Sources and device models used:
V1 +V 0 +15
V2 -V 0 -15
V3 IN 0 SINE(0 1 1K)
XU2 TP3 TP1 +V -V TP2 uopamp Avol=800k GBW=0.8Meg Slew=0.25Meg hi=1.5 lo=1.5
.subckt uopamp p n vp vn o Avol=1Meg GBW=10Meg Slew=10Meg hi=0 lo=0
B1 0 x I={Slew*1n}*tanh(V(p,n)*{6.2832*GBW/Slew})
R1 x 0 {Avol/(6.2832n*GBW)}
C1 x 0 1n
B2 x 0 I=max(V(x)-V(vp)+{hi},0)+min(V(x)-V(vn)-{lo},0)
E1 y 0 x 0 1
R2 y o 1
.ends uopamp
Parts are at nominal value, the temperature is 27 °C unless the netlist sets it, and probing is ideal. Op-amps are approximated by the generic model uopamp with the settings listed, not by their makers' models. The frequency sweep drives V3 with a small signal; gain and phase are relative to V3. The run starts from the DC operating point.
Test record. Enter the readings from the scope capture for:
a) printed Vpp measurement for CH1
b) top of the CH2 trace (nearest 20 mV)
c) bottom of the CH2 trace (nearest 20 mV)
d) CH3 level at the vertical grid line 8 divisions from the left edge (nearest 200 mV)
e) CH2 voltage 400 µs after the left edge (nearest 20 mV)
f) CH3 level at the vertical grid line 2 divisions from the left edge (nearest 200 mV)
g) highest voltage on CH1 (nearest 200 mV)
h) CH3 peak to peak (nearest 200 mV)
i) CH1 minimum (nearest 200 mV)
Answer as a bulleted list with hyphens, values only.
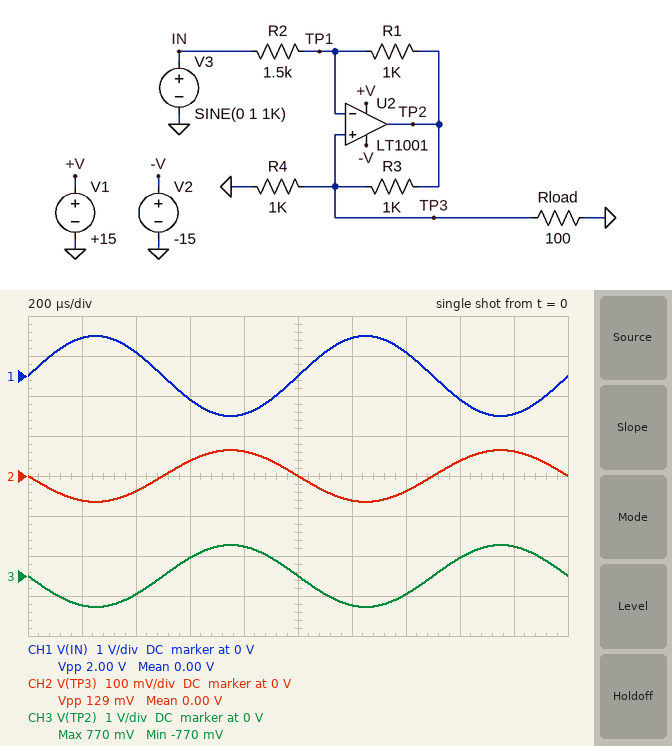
- 2.00 V
- 60 mV
- -60 mV
- 400 mV
- -40 mV
- -400 mV
- 1.0 V
- 1.6 V
- -1.0 V
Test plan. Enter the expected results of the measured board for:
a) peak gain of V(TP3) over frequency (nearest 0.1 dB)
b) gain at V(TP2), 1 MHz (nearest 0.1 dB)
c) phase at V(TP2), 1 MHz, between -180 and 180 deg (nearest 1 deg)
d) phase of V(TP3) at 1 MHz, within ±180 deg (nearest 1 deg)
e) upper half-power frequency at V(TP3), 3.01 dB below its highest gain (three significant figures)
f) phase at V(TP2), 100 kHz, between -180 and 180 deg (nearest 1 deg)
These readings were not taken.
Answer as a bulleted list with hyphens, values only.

- -23.8 dB
- -10.6 dB
- 112 deg
- 112 deg
- 413 kHz
- 166 deg
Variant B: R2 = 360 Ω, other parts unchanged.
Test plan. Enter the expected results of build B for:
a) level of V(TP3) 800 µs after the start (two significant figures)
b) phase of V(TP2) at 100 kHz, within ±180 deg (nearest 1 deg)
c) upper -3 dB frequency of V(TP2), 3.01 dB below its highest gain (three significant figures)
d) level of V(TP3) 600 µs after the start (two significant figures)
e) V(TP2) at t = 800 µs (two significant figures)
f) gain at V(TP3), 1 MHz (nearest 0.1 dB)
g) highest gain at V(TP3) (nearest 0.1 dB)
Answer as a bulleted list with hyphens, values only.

- 320 mV
- 145 deg
- 145 kHz
- 200 mV
- 3.9 V
- -26.3 dB
- -9.4 dB
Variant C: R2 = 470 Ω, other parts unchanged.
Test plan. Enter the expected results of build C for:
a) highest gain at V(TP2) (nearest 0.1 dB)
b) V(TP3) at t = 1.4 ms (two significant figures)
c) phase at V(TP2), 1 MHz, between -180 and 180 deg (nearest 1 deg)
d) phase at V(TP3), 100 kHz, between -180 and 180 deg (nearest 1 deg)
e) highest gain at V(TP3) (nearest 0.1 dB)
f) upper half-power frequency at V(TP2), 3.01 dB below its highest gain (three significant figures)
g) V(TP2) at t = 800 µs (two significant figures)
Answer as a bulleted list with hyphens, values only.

- 9.2 dB
- -140 mV
- 101 deg
- 152 deg
- -12.4 dB
- 189 kHz
- 2.7 V
